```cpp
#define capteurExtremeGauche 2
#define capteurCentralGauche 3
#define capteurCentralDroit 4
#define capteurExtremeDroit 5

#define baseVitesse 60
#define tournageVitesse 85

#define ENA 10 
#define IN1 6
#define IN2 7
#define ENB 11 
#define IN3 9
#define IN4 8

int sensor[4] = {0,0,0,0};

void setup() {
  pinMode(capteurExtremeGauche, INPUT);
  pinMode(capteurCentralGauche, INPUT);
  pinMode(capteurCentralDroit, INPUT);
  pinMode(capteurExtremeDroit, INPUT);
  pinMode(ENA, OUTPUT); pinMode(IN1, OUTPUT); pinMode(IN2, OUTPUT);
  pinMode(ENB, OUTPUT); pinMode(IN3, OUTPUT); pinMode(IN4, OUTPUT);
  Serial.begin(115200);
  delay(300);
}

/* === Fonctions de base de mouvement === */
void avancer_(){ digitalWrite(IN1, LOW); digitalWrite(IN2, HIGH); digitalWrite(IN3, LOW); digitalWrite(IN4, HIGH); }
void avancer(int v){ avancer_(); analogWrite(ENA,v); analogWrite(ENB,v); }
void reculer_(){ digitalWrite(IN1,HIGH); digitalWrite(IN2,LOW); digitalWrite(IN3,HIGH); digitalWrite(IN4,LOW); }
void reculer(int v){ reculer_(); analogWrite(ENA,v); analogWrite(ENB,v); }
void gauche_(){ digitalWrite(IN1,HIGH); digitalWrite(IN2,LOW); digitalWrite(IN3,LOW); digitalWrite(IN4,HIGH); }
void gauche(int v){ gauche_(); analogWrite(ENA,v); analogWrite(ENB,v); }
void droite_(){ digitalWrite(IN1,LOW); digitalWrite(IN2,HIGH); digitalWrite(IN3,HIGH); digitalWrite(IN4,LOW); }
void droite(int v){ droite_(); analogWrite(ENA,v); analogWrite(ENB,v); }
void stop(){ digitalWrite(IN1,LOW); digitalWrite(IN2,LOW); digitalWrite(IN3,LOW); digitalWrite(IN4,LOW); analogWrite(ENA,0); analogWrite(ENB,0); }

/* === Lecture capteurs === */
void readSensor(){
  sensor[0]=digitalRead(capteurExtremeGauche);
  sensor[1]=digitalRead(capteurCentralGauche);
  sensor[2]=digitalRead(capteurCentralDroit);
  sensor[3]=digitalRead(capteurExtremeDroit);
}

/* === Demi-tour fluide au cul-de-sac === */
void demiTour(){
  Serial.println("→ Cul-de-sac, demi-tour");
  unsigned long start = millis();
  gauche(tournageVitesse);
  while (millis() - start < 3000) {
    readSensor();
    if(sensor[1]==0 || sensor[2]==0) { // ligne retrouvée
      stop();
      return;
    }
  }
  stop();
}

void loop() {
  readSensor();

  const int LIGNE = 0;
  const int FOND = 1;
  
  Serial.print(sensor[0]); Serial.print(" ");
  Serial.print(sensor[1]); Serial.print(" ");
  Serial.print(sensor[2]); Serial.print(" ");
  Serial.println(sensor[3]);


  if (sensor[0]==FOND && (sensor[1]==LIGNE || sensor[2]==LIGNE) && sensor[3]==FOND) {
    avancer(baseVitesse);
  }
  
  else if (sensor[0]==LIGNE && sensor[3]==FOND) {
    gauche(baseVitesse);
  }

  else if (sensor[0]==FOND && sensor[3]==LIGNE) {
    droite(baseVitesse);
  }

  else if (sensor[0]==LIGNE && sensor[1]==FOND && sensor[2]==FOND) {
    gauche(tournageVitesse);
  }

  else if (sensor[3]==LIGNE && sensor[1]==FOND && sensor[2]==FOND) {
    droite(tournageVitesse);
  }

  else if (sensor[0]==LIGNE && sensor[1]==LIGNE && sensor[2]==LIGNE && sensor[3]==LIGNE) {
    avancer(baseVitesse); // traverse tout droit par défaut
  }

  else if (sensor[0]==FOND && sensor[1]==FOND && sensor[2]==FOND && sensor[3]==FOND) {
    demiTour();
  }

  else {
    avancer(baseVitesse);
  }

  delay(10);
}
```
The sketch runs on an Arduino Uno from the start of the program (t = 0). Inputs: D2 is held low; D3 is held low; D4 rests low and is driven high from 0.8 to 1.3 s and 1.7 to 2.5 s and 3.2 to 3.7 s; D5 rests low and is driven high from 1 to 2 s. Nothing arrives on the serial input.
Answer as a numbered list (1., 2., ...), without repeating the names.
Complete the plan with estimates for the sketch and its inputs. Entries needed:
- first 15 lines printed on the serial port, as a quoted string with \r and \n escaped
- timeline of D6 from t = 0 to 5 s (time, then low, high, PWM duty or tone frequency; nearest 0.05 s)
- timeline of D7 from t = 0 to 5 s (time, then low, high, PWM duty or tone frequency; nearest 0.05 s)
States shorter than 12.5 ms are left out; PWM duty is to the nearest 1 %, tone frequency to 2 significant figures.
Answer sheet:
1. "0 0 0 0\r\n0 0 0 0\r\n0 0 0 0\r\n0 0 0 0\r\n0 0 0 0\r\n0 0 0 0\r\n0 0 0 0\r\n0 0 0 0\r\n0 0 0 0\r\n0 0 0 0\r\n0 0 0 0\r\n0 0 0 0\r\n0 0 0 0\r\n0 0 0 0\r\n0 0 0 0\r\n"
2. 0 s low; 1 s high; 2 s low
3. 0 s low; 0.3 s high; 1 s low; 2 s high
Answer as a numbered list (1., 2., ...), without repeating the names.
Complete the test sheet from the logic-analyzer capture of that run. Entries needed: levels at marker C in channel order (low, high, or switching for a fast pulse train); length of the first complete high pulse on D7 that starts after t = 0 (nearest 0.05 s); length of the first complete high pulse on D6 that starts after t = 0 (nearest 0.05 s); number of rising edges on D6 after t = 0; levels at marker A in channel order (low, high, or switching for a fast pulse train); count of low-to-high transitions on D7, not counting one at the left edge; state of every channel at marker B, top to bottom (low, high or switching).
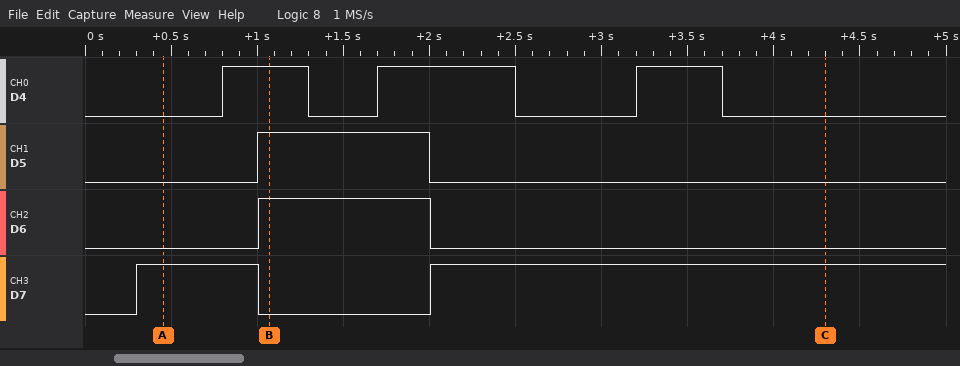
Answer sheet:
1. D4 low, D5 low, D6 low, D7 high
2. 0.70 s
3. 1.00 s
4. 1
5. D4 low, D5 low, D6 low, D7 high
6. 2
7. D4 high, D5 high, D6 high, D7 low
